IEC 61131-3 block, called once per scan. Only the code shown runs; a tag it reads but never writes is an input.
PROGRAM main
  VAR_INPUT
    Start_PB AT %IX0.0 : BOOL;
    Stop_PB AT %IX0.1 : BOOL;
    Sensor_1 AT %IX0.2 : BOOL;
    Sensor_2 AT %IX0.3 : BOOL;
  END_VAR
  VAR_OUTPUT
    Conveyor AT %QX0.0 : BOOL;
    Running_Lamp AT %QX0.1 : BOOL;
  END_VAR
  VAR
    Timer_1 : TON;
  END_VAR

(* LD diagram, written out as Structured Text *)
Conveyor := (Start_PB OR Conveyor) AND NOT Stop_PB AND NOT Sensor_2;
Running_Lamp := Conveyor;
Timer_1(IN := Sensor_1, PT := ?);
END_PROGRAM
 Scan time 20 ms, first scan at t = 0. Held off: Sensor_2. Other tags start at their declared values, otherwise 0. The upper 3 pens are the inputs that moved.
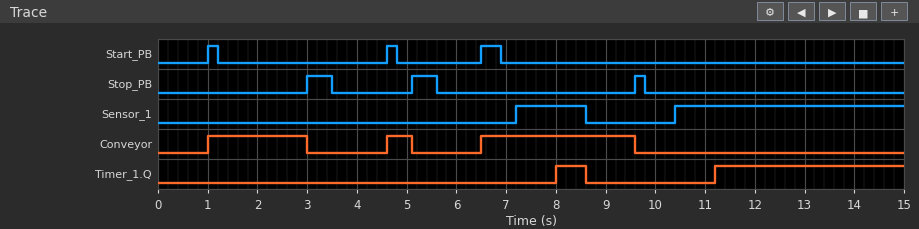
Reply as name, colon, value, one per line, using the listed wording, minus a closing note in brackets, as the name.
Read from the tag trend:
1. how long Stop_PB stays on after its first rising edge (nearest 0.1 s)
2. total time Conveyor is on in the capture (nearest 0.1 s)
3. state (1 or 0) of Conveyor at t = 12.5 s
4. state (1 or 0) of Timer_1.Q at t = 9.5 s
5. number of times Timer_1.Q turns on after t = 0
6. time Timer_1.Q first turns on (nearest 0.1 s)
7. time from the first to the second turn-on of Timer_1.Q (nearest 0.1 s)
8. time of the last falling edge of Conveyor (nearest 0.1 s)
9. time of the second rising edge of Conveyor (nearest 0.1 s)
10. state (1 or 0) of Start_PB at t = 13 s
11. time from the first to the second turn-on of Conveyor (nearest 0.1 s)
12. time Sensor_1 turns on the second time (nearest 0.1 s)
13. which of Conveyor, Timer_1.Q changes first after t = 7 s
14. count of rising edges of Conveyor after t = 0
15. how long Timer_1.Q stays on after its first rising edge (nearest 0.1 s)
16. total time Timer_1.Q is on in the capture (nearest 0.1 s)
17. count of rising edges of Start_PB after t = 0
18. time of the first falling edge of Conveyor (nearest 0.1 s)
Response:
how long Stop_PB stays on after its first rising edge: 0.5 s
total time Conveyor is on in the capture: 5.6 s
state (1 or 0) of Conveyor at t = 12.5 s: 0
state (1 or 0) of Timer_1.Q at t = 9.5 s: 0
number of times Timer_1.Q turns on after t = 0: 2
time Timer_1.Q first turns on: 8.0 s
time from the first to the second turn-on of Timer_1.Q: 3.2 s
time of the last falling edge of Conveyor: 9.6 s
time of the second rising edge of Conveyor: 4.6 s
state (1 or 0) of Start_PB at t = 13 s: 0
time from the first to the second turn-on of Conveyor: 3.6 s
time Sensor_1 turns on the second time: 10.4 s
which of Conveyor, Timer_1.Q changes first after t = 7 s: Timer_1.Q
count of rising edges of Conveyor after t = 0: 3
how long Timer_1.Q stays on after its first rising edge: 0.6 s
total time Timer_1.Q is on in the capture: 4.4 s
count of rising edges of Start_PB after t = 0: 3
time of the first falling edge of Conveyor: 3.0 s
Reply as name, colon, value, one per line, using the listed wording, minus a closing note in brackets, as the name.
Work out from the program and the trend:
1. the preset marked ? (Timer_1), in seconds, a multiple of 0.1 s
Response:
the preset marked ? (Timer_1), in seconds, a multiple of 0.1 s: 0.8 s
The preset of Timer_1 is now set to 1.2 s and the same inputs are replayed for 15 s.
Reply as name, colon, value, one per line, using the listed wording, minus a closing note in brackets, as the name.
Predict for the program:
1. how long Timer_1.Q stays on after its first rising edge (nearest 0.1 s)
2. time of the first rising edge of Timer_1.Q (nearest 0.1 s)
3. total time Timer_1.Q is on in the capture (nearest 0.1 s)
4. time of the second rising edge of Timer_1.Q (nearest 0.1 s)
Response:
how long Timer_1.Q stays on after its first rising edge: 0.2 s
time of the first rising edge of Timer_1.Q: 8.4 s
total time Timer_1.Q is on in the capture: 3.6 s
time of the second rising edge of Timer_1.Q: 11.6 s
